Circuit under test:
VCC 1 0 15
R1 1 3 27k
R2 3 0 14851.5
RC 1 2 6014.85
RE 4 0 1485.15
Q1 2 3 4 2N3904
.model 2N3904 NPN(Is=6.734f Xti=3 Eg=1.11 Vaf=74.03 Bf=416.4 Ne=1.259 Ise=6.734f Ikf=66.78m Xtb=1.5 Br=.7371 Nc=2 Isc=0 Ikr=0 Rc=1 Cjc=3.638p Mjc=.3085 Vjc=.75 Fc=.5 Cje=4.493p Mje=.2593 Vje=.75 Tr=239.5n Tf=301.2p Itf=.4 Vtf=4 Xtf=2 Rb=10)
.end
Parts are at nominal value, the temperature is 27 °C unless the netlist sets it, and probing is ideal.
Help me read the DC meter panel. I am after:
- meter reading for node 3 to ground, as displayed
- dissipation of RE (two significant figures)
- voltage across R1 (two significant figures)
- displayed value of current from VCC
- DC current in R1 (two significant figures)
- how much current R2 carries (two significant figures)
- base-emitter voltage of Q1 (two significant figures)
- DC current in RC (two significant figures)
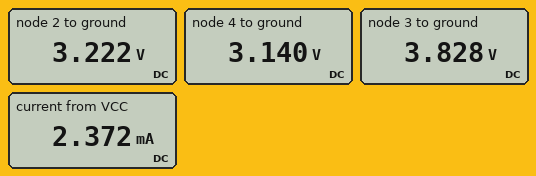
3.828 V
6.6 mW
11 V
2.372 mA
410 µA
260 µA
690 mV
2.0 mA
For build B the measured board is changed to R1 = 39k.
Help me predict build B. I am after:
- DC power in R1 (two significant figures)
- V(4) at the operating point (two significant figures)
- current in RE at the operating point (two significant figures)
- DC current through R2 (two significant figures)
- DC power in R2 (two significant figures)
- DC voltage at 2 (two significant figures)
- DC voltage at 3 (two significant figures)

3.3 mW
3.0 V
2.0 mA
250 µA
910 µW
3.1 V
3.7 V
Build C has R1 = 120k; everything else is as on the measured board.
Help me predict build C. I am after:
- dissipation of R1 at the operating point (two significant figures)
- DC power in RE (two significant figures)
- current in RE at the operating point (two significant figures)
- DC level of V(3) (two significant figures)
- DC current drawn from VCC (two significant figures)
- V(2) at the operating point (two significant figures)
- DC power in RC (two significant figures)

1.5 mW
600 µW
630 µA
1.6 V
740 µA
11 V
2.4 mW
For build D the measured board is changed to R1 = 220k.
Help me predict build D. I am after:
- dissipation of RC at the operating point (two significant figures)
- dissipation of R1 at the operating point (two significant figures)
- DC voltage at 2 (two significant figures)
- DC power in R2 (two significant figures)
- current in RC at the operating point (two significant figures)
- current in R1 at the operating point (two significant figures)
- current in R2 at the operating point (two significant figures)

250 µW
900 µW
14 V
58 µW
200 µA
64 µA
62 µA
